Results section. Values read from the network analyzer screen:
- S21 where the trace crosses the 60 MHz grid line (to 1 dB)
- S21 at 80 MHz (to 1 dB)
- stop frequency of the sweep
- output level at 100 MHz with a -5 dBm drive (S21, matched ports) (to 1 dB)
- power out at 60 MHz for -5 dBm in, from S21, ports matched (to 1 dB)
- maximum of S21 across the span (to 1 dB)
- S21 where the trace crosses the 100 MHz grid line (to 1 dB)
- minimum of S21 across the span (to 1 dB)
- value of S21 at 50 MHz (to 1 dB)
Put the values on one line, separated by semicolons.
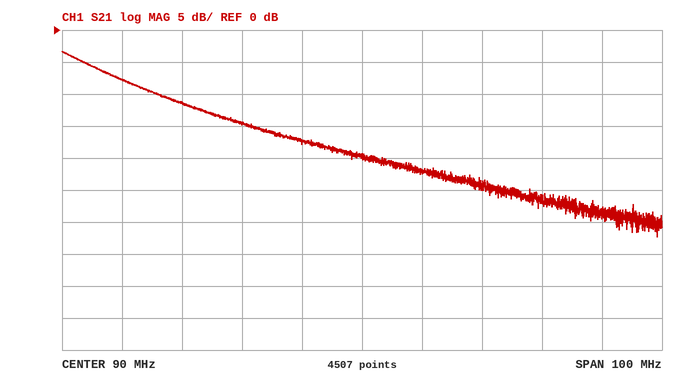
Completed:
-11 dB; -17 dB; 140 MHz; -27 dBm; -16 dBm; -3 dB; -22 dB; -32 dB; -8 dB
